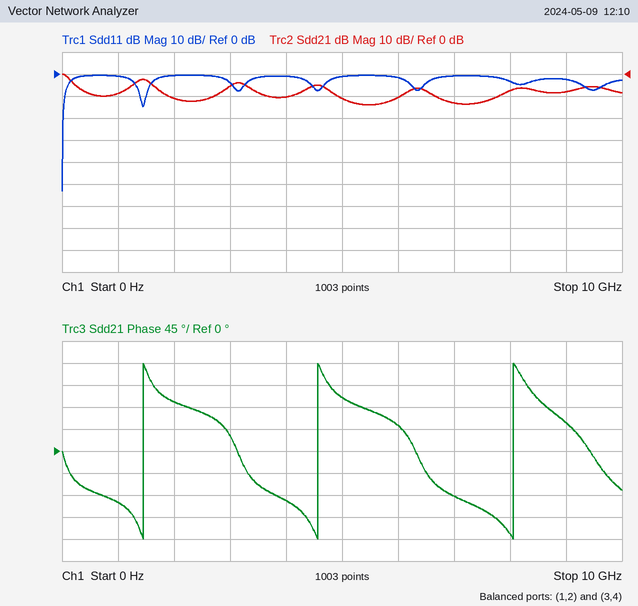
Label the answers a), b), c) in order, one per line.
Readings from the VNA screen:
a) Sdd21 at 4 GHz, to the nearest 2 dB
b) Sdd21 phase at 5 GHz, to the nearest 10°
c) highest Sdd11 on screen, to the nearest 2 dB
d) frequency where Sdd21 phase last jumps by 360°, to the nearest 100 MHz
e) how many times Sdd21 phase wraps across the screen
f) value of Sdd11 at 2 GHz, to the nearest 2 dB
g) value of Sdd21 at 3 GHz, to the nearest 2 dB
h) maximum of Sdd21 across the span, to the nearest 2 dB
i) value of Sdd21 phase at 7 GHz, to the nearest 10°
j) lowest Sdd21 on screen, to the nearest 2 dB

a) -10 dB
b) 110°
c) 0 dB
d) 8.1 GHz
e) 3
f) 0 dB
g) -6 dB
h) 0 dB
i) -90°
j) -14 dB
